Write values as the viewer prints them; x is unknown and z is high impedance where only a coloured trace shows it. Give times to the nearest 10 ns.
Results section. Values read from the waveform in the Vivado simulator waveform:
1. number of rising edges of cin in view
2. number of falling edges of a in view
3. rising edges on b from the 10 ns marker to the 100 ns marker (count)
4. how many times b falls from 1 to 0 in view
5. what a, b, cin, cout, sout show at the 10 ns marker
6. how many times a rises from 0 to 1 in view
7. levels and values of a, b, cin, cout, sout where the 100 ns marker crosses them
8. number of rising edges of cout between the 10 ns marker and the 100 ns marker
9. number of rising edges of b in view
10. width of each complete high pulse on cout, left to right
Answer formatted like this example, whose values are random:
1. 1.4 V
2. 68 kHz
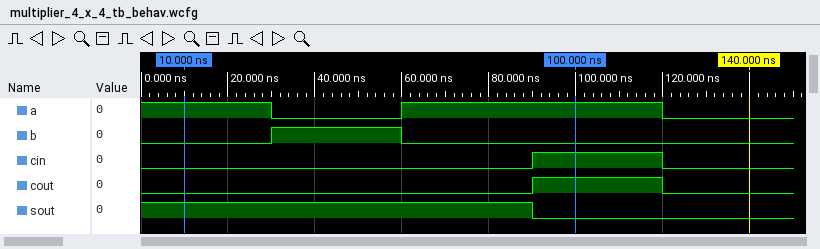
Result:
1. 1
2. 2
3. 1
4. 1
5. a=1, b=0, cin=0, cout=0, sout=1
6. 1
7. a=1, b=0, cin=1, cout=1, sout=0
8. 1
9. 1
10. 30 ns
